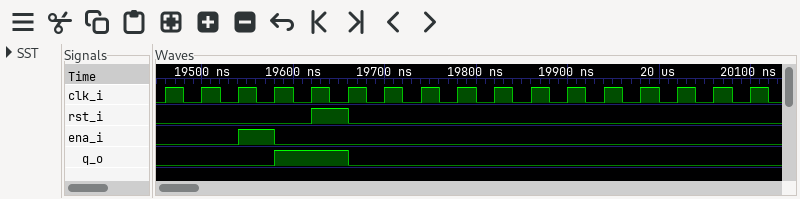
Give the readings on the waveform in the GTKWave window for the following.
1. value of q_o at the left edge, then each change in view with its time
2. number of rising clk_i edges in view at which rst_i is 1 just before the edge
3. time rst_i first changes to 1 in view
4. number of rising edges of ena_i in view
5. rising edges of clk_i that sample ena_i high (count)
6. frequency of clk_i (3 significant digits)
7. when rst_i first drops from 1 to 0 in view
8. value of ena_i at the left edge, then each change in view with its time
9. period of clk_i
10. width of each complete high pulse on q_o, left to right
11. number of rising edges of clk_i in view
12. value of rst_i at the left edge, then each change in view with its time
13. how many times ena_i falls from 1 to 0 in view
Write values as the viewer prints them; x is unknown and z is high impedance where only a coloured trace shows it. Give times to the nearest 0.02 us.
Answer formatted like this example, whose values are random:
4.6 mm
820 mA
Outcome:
0, 1 at 19.58 us, 0 at 19.66 us
1
19.62 us
1
1
25.0 MHz
19.66 us
0, 1 at 19.54 us, 0 at 19.58 us
0.04 us
0.08 us
17
0, 1 at 19.62 us, 0 at 19.66 us
1
